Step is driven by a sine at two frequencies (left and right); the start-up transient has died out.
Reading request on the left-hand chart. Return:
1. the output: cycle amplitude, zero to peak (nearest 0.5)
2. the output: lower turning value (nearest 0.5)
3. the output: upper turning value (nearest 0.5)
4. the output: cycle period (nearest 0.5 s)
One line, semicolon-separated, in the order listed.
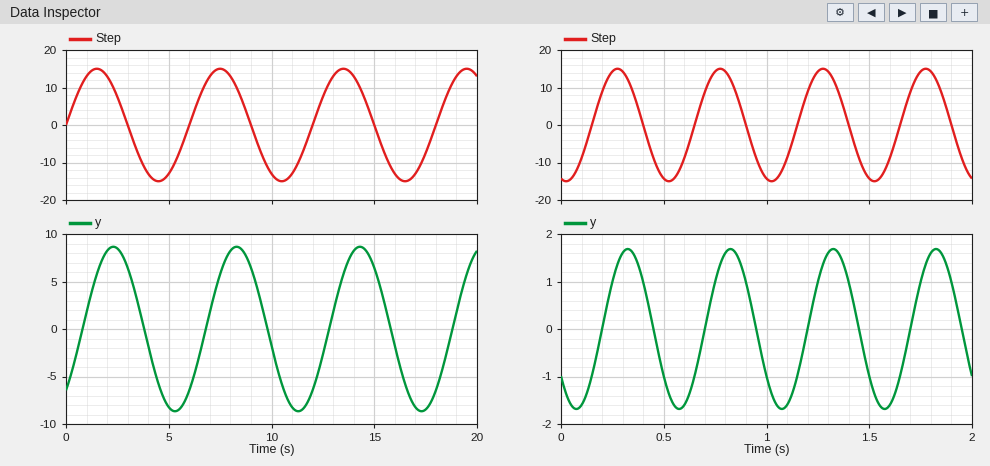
8.5; -8.5; 8.5; 6.0 s
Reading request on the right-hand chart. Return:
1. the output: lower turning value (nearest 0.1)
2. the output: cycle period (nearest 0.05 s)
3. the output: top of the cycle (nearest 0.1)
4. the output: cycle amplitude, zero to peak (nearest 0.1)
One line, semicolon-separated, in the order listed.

-1.7; 0.50 s; 1.7; 1.7
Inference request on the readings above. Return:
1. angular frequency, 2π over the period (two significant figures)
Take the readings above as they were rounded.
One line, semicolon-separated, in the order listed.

13 rad/s
